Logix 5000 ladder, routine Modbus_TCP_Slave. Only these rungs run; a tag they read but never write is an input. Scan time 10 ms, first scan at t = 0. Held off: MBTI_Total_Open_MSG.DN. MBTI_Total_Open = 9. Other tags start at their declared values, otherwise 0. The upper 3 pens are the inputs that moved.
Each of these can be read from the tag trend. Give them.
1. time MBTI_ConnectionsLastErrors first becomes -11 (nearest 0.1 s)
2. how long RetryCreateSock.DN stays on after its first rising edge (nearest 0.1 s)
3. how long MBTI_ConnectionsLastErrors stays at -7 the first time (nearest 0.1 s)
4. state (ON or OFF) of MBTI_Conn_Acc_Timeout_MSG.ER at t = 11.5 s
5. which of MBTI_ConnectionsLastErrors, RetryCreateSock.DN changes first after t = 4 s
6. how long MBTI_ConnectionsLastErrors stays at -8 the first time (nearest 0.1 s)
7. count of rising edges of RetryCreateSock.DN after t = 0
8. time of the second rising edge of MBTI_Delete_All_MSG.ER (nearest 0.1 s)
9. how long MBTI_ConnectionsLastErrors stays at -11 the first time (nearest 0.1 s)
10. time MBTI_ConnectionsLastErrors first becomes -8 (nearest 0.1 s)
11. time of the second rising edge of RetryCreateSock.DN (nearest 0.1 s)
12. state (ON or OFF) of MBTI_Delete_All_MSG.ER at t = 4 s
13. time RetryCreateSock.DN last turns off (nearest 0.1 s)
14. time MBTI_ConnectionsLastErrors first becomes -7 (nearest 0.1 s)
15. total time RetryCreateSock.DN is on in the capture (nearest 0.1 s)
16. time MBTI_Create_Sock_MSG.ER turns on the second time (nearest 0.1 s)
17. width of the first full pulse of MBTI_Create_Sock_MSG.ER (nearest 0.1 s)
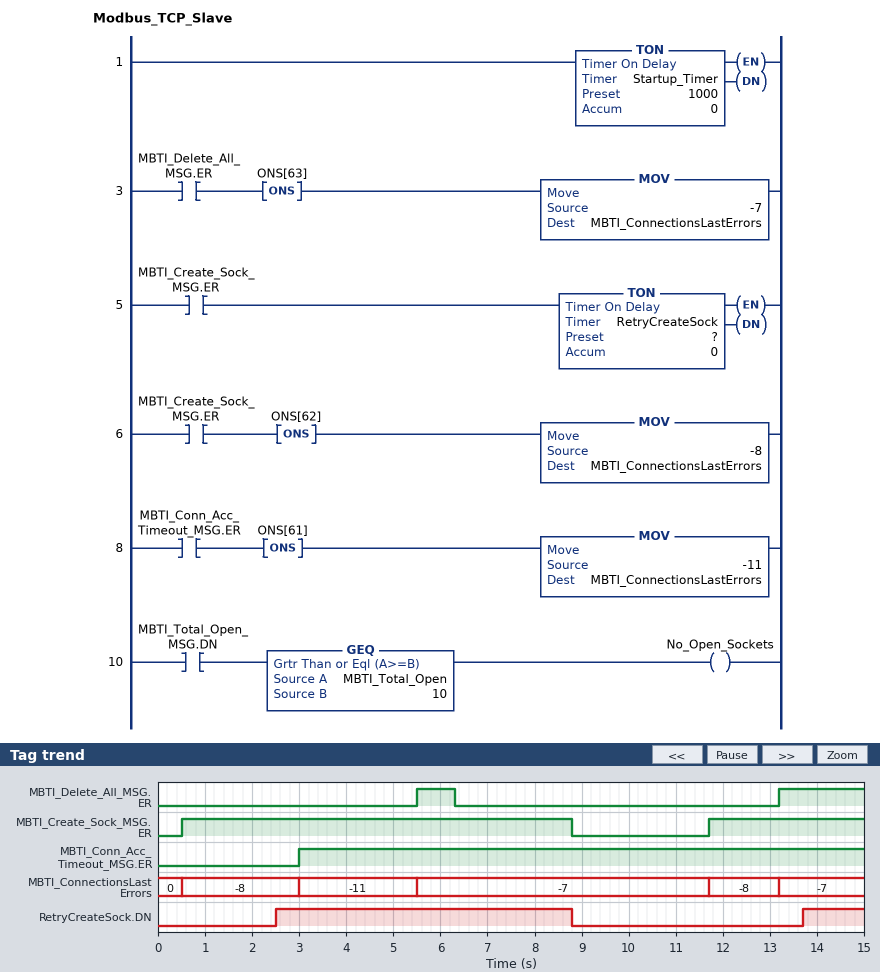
3.0 s
6.3 s
6.2 s
ON
MBTI_ConnectionsLastErrors
2.5 s
2
13.2 s
2.5 s
0.5 s
13.7 s
OFF
8.8 s
5.5 s
7.6 s
11.7 s
8.3 s
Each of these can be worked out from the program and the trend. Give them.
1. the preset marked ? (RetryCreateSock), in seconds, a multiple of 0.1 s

2.0 s
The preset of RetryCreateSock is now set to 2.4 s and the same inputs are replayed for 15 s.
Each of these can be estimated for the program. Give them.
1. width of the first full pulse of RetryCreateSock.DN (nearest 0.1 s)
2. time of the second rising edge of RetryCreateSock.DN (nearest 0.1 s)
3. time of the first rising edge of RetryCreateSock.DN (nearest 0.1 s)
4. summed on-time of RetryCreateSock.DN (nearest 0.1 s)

5.9 s
14.1 s
2.9 s
6.8 s
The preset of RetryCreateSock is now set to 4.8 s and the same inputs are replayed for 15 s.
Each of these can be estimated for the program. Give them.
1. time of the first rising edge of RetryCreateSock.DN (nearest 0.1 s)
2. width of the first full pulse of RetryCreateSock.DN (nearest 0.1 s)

5.3 s
3.5 s
